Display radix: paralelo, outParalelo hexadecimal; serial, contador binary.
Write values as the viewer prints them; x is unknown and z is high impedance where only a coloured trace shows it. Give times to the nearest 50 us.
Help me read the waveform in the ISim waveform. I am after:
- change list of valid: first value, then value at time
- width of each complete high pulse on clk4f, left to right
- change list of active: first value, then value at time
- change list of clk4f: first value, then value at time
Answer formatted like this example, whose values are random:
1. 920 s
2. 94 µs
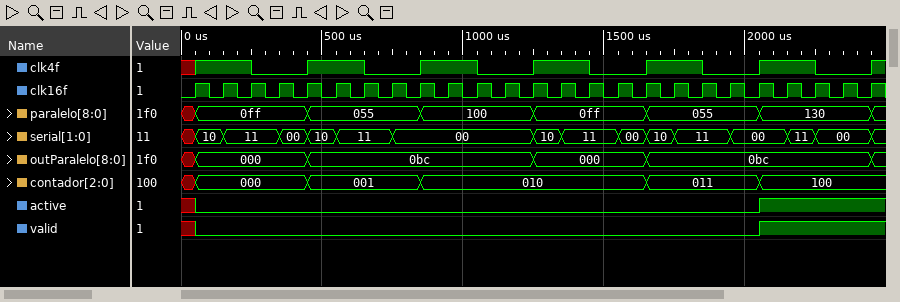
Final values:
1. x, 0 at 50 us, 1 at 2050 us
2. 200 us, 200 us, 200 us, 200 us, 200 us
3. x, 0 at 50 us, 1 at 2050 us
4. x, 1 at 50 us, 0 at 250 us, 1 at 450 us, 0 at 650 us, 1 at 850 us, 0 at 1050 us, 1 at 1250 us, 0 at 1450 us, 1 at 1650 us, 0 at 1850 us, 1 at 2050 us, 0 at 2250 us, 1 at 2450 us
